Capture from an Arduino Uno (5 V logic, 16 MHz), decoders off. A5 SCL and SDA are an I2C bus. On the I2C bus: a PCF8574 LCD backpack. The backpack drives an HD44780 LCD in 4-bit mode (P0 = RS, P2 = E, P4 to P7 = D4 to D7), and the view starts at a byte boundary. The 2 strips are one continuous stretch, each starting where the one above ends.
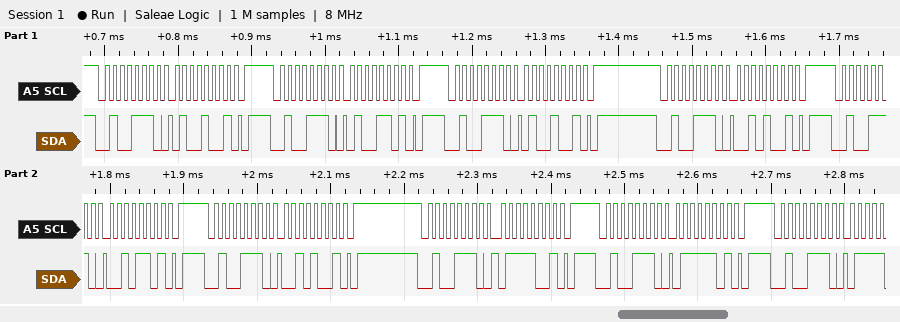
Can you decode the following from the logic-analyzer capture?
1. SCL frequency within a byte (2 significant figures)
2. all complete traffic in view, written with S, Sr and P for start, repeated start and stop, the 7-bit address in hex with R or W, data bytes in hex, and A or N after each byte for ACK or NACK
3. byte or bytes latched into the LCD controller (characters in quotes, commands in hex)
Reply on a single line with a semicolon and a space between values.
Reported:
100 kHz; S 27W A 49 A P S 27W A 4D A P S 27W A 49 A P S 27W A 29 A P S 27W A 2D A P S 27W A 29 A P S 27W A 79 A P S 27W A 7D A P S 27W A; 'B'
